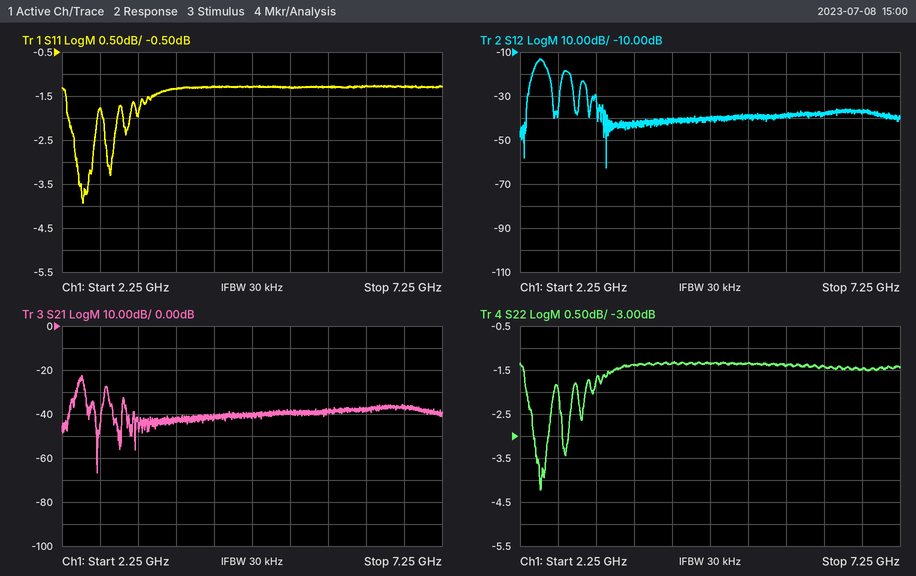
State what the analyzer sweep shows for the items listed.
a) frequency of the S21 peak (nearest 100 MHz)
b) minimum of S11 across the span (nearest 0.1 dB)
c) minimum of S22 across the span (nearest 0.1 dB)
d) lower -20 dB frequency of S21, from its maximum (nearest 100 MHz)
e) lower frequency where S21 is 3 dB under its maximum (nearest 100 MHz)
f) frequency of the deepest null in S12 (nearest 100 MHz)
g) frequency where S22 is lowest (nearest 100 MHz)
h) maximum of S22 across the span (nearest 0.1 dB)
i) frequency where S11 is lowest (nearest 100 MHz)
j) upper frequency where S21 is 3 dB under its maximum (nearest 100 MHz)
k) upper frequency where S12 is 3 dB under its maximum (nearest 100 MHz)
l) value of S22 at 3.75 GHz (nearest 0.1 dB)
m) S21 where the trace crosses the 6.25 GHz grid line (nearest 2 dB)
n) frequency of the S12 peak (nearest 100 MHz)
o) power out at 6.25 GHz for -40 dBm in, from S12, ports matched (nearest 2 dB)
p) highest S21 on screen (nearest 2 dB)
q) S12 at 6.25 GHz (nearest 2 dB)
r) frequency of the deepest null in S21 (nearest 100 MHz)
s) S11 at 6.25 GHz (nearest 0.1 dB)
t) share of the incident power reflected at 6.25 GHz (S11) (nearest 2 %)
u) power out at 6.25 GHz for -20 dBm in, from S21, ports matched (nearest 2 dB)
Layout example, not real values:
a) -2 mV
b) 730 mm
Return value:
a) 2.5 GHz
b) -3.9 dB
c) -4.2 dB
d) 2.3 GHz
e) 2.5 GHz
f) 3.4 GHz
g) 2.5 GHz
h) -1.3 dB
i) 2.5 GHz
j) 2.5 GHz
k) 2.6 GHz
l) -1.4 dB
m) -38 dB
n) 2.5 GHz
o) -78 dBm
p) -22 dB
q) -38 dB
r) 2.7 GHz
s) -1.3 dB
t) 74 %
u) -58 dBm
